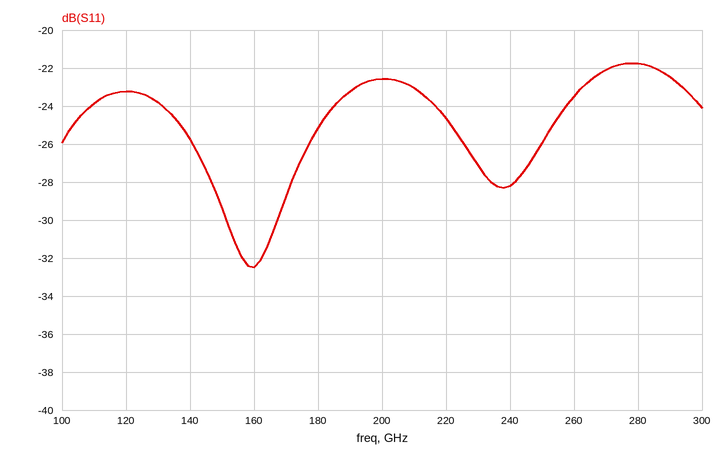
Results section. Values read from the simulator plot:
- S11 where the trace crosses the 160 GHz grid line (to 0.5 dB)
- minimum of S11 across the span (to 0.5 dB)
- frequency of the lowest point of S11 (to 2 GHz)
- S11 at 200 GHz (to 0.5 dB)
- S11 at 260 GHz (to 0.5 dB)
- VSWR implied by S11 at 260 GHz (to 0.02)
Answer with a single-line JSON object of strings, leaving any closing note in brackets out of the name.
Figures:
{"S11 where the trace crosses the 160 GHz grid line": "-32.5 dB", "minimum of S11 across the span": "-32.5 dB", "frequency of the lowest point of S11": "160 GHz", "S11 at 200 GHz": "-22.5 dB", "S11 at 260 GHz": "-23.5 dB", "VSWR implied by S11 at 260 GHz": "1.14"}
